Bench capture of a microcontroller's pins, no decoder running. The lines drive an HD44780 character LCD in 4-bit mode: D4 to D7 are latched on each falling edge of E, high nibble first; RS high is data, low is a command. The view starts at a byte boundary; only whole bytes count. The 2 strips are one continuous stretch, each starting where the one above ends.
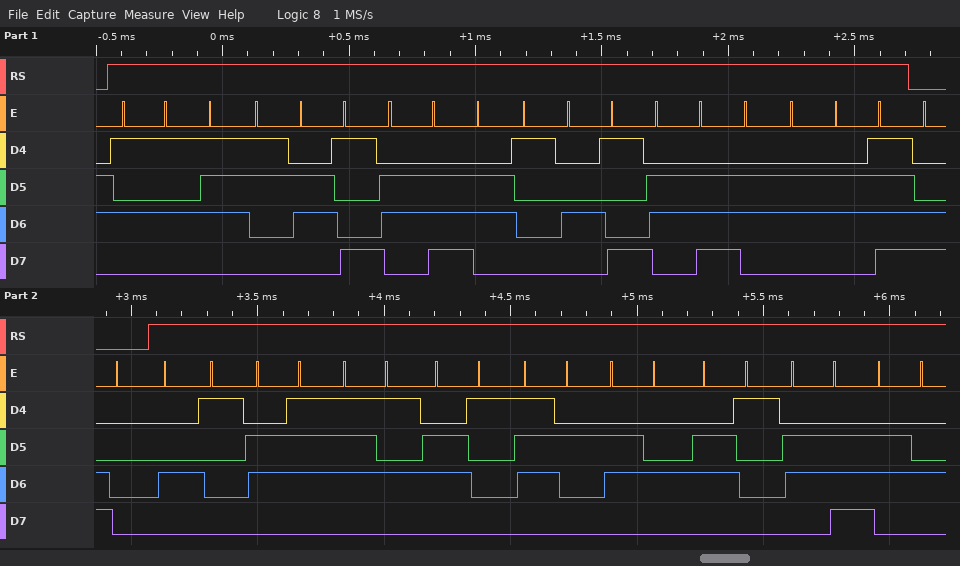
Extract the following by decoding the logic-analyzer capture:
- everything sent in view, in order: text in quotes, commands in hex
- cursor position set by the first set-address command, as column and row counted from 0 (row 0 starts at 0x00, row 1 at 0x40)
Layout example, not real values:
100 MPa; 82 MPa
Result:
"UsinaInfo" 0xC0 "Aguardand"; column 0, row 1
